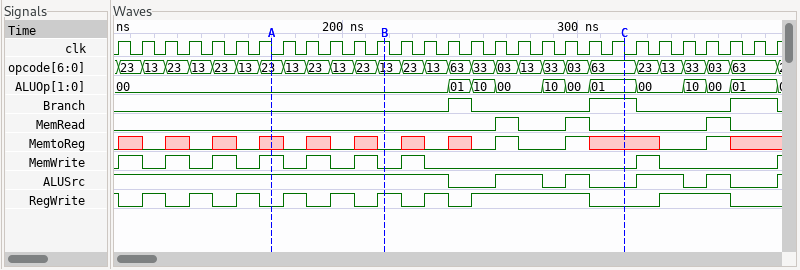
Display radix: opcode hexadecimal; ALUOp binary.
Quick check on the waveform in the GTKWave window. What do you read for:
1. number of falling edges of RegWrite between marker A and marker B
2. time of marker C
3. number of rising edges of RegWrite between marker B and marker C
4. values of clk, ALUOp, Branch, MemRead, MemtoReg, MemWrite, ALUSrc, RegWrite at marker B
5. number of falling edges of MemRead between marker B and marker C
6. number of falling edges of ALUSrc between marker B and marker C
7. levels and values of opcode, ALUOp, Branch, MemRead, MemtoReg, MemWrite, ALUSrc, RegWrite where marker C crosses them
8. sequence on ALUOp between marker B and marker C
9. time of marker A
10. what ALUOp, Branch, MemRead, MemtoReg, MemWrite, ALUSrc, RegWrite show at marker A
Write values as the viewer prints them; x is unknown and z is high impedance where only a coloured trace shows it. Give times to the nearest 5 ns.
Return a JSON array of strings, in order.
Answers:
["2", "320 ns", "2", "clk=1, ALUOp=00, Branch=0, MemRead=0, MemtoReg=0, MemWrite=0, ALUSrc=1, RegWrite=1", "2", "3", "opcode=63, ALUOp=01, Branch=1, MemRead=0, MemtoReg=x, MemWrite=0, ALUSrc=0, RegWrite=0", "00, 01, 10, 00, 10, 00, 01", "170 ns", "ALUOp=00, Branch=0, MemRead=0, MemtoReg=x, MemWrite=1, ALUSrc=1, RegWrite=0"]
